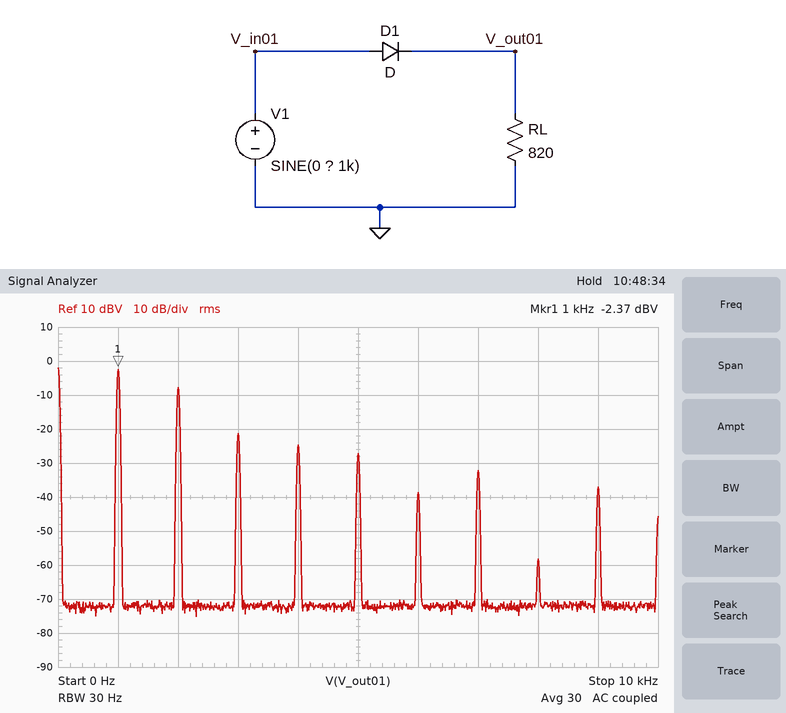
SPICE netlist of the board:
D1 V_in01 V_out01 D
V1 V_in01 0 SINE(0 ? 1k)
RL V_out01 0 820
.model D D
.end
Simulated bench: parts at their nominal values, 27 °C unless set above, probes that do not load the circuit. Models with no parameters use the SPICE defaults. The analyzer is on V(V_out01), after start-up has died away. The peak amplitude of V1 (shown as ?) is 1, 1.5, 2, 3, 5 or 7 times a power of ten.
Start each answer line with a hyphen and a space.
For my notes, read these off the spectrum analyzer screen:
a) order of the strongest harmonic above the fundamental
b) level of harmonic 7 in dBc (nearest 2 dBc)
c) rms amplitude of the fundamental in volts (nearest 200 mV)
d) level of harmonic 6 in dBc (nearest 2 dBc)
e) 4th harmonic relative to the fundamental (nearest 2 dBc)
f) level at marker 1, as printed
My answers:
- 2
- -30 dBc
- 800 mV
- -36 dBc
- -22 dBc
- -2.37 dBV
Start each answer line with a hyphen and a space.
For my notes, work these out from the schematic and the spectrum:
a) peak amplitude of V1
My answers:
- 3 V
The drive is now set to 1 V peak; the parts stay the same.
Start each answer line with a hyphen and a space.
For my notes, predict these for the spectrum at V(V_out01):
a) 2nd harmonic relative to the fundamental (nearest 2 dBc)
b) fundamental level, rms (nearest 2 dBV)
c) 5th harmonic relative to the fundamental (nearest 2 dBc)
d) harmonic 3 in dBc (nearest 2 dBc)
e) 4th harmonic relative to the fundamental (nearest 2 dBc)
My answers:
- -2 dBc
- -20 dBV
- -36 dBc
- -8 dBc
- -16 dBc
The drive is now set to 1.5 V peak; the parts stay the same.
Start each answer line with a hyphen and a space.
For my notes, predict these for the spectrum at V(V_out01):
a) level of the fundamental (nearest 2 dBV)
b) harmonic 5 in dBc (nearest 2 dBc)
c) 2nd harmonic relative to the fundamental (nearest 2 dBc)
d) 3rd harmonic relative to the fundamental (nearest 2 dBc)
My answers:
- -12 dBV
- -22 dBc
- -4 dBc
- -12 dBc
